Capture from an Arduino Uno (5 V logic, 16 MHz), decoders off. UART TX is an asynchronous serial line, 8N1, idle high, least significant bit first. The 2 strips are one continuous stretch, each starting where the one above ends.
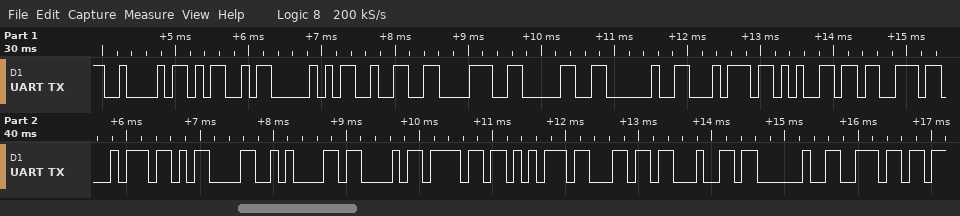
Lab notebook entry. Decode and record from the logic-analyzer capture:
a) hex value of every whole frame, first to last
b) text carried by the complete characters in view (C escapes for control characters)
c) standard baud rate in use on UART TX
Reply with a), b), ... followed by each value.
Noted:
a) 0x42 0x4D 0x50 0x32 0x38 0x30 0x20 0x74 0x65 0x73 0x74 0x0D 0x0A 0x43 0x6F 0x75 0x6C 0x64 0x20 0x6E
b) "BMP280 test\r\nCould n"
c) 9600 baud
